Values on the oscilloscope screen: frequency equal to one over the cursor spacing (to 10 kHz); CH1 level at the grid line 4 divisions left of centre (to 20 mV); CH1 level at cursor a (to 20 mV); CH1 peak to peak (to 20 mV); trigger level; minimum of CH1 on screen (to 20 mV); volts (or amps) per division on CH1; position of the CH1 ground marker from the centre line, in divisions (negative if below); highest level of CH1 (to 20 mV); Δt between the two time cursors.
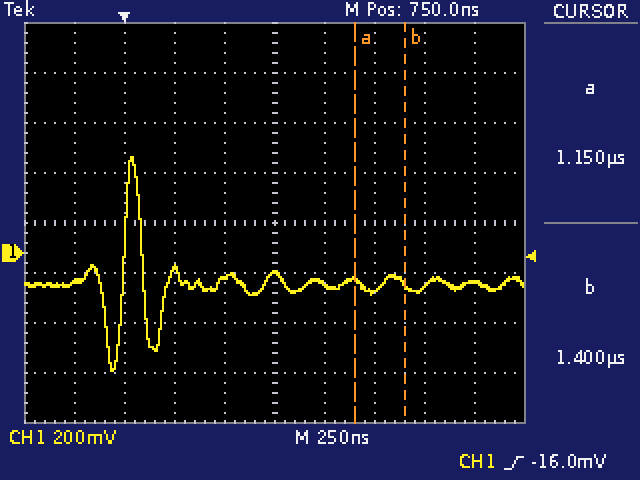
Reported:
4.00 MHz
-120 mV
-120 mV
860 mV
-16.0 mV
-480 mV
200 mV
-0.6 div
380 mV
250 ns
